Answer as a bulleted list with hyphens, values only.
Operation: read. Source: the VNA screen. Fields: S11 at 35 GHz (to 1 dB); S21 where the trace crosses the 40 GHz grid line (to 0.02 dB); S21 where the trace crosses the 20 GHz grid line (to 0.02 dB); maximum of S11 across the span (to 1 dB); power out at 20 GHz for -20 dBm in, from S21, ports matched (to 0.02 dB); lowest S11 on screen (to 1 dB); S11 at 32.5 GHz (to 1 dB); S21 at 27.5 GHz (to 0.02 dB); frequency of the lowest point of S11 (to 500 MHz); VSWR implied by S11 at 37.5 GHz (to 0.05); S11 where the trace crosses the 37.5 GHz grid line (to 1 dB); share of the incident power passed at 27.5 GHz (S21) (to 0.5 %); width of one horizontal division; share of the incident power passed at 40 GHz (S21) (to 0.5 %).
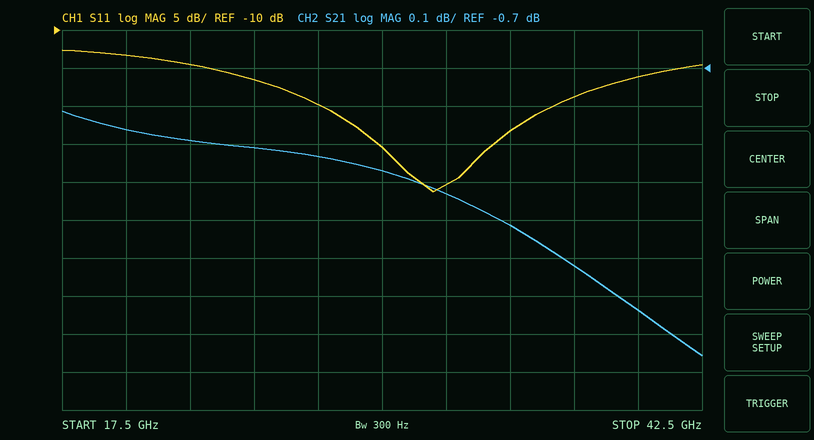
- -23 dB
- -1.34 dB
- -0.86 dB
- -13 dB
- -20.86 dBm
- -31 dB
- -30 dB
- -0.94 dB
- 32.0 GHz
- 1.25
- -19 dB
- 80.5 %
- 2.5 GHz
- 73.5 %
